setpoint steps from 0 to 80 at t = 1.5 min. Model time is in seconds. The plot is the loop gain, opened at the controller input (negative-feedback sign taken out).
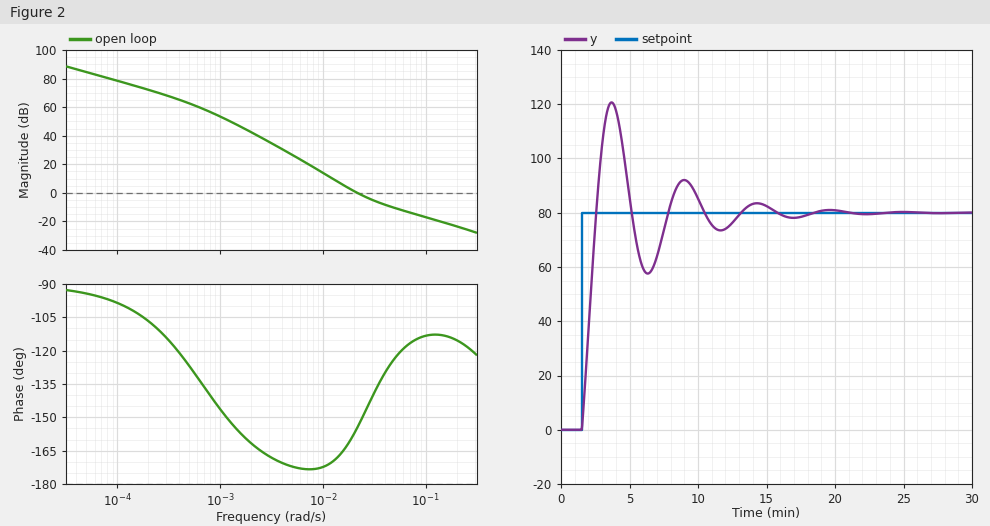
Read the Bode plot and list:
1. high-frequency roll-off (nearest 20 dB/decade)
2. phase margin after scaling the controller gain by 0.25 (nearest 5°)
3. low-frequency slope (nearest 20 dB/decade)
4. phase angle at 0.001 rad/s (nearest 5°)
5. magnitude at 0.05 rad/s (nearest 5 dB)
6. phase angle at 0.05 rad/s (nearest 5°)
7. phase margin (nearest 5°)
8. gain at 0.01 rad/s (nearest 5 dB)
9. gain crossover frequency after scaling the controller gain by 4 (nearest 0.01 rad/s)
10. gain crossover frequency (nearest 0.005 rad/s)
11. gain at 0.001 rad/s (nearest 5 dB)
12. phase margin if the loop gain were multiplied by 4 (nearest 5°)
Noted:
-20 dB/decade
10°
-20 dB/decade
-145°
-10 dB
-125°
25°
15 dB
0.06 rad/s
0.020 rad/s
55 dB
60°
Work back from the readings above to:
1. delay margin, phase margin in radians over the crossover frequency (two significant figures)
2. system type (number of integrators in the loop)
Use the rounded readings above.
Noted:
22 s
1
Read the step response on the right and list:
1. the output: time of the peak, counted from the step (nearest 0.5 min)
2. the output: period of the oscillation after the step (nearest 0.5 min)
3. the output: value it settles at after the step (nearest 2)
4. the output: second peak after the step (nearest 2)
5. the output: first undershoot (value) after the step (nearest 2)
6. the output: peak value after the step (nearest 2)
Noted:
2.0 min
5.5 min
80
92
58
120
